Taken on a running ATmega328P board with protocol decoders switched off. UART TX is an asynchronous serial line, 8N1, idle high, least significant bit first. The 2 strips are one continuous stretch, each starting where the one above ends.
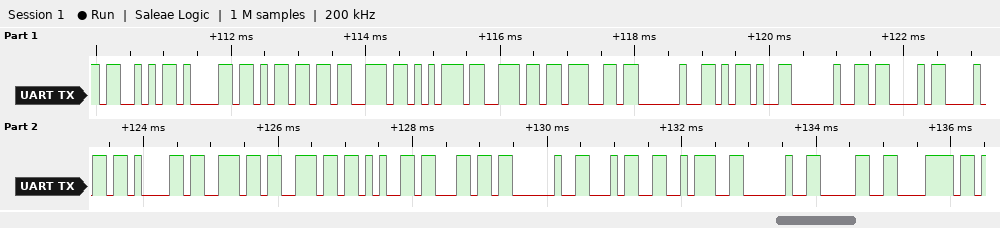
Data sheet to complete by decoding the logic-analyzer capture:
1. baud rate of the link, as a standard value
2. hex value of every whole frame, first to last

9600 baud
53 61 6D 73 75 6E 67 20 2D 20 43 68 61 6E 6E 65 6C 20 34 3A 20 30 78
